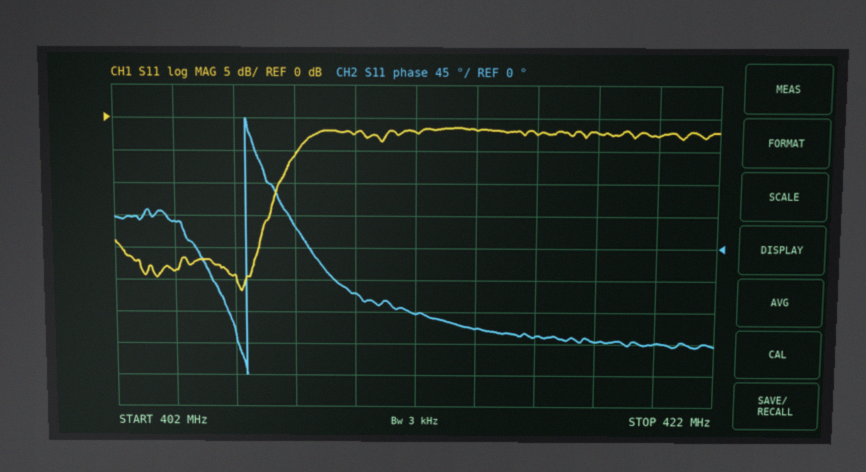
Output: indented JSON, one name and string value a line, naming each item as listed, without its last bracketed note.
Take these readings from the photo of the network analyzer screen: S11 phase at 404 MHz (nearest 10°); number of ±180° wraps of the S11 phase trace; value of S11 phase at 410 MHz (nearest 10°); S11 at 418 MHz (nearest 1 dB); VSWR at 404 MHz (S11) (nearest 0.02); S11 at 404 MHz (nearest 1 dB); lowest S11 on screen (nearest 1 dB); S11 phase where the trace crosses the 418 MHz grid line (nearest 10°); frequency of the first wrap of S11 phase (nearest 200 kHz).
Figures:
{
  "S11 phase at 404 MHz": "40°",
  "number of ±180° wraps of the S11 phase trace": "1",
  "value of S11 phase at 410 MHz": "-60°",
  "S11 at 418 MHz": "-2 dB",
  "VSWR at 404 MHz (S11)": "1.14",
  "S11 at 404 MHz": "-24 dB",
  "lowest S11 on screen": "-27 dB",
  "S11 phase where the trace crosses the 418 MHz grid line": "-130°",
  "frequency of the first wrap of S11 phase": "406.4 MHz"
}
